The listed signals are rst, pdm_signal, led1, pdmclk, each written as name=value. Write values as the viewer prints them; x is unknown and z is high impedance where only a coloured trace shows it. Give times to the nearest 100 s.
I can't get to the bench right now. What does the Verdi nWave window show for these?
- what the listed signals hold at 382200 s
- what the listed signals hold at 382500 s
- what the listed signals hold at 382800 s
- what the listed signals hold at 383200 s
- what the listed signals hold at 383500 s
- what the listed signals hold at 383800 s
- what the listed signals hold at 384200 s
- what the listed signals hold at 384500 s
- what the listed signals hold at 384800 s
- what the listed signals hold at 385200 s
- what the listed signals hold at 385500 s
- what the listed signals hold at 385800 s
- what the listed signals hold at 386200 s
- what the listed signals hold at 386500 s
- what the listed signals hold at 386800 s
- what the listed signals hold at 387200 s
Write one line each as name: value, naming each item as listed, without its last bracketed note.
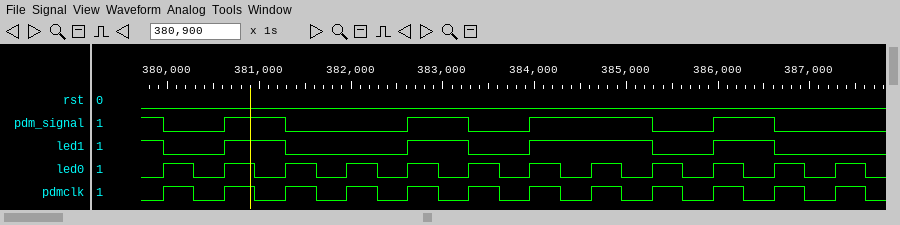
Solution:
what the listed signals hold at 382200 s: rst=0, pdm_signal=0, led1=0, pdmclk=1
what the listed signals hold at 382500 s: rst=0, pdm_signal=0, led1=0, pdmclk=0
what the listed signals hold at 382800 s: rst=0, pdm_signal=1, led1=1, pdmclk=1
what the listed signals hold at 383200 s: rst=0, pdm_signal=1, led1=1, pdmclk=0
what the listed signals hold at 383500 s: rst=0, pdm_signal=0, led1=0, pdmclk=1
what the listed signals hold at 383800 s: rst=0, pdm_signal=0, led1=0, pdmclk=0
what the listed signals hold at 384200 s: rst=0, pdm_signal=1, led1=1, pdmclk=1
what the listed signals hold at 384500 s: rst=0, pdm_signal=1, led1=1, pdmclk=0
what the listed signals hold at 384800 s: rst=0, pdm_signal=1, led1=1, pdmclk=1
what the listed signals hold at 385200 s: rst=0, pdm_signal=1, led1=1, pdmclk=0
what the listed signals hold at 385500 s: rst=0, pdm_signal=0, led1=0, pdmclk=1
what the listed signals hold at 385800 s: rst=0, pdm_signal=0, led1=0, pdmclk=0
what the listed signals hold at 386200 s: rst=0, pdm_signal=1, led1=1, pdmclk=1
what the listed signals hold at 386500 s: rst=0, pdm_signal=1, led1=1, pdmclk=0
what the listed signals hold at 386800 s: rst=0, pdm_signal=0, led1=0, pdmclk=1
what the listed signals hold at 387200 s: rst=0, pdm_signal=0, led1=0, pdmclk=0
